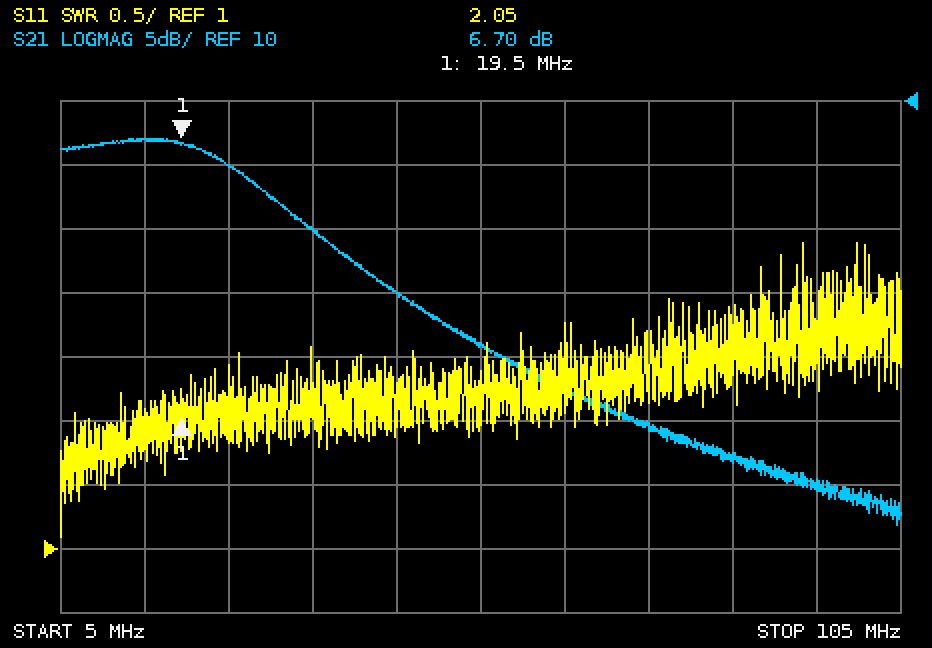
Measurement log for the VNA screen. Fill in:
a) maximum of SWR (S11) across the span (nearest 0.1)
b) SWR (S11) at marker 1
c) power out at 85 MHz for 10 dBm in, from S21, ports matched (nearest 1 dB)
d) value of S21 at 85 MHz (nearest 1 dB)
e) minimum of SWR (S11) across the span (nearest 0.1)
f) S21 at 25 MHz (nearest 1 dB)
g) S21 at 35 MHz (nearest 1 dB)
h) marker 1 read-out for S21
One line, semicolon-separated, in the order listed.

3.4; 2.05; -8 dBm; -18 dB; 1.1; 5 dB; 0 dB; 6.70 dB
